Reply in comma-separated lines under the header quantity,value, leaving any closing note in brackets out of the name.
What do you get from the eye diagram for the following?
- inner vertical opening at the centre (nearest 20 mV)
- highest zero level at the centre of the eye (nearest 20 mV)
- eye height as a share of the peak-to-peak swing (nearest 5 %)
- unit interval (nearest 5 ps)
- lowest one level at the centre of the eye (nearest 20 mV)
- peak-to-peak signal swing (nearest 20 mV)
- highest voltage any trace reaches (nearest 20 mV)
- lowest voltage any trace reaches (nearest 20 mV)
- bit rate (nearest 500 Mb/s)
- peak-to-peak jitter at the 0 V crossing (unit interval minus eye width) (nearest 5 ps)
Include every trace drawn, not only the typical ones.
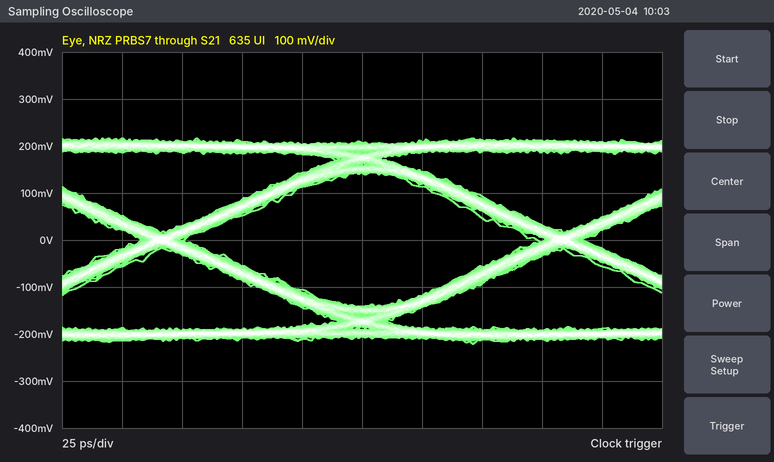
quantity,value
inner vertical opening at the centre,280 mV
highest zero level at the centre of the eye,-140 mV
eye height as a share of the peak-to-peak swing,65 %
unit interval,165 ps
lowest one level at the centre of the eye,140 mV
peak-to-peak signal swing,440 mV
highest voltage any trace reaches,220 mV
lowest voltage any trace reaches,-220 mV
bit rate,6.0 Gb/s
peak-to-peak jitter at the 0 V crossing (unit interval minus eye width),20 ps
